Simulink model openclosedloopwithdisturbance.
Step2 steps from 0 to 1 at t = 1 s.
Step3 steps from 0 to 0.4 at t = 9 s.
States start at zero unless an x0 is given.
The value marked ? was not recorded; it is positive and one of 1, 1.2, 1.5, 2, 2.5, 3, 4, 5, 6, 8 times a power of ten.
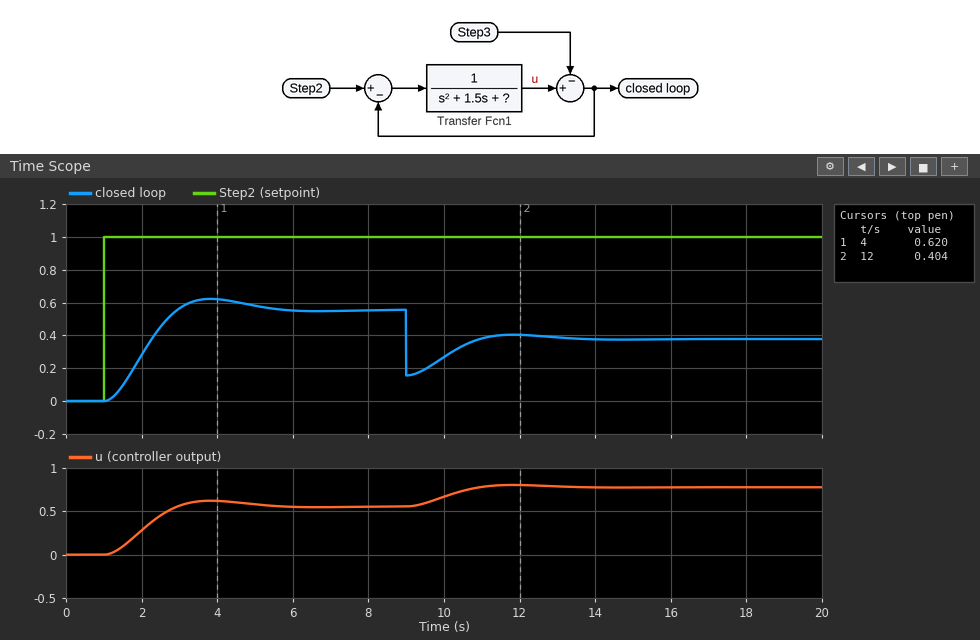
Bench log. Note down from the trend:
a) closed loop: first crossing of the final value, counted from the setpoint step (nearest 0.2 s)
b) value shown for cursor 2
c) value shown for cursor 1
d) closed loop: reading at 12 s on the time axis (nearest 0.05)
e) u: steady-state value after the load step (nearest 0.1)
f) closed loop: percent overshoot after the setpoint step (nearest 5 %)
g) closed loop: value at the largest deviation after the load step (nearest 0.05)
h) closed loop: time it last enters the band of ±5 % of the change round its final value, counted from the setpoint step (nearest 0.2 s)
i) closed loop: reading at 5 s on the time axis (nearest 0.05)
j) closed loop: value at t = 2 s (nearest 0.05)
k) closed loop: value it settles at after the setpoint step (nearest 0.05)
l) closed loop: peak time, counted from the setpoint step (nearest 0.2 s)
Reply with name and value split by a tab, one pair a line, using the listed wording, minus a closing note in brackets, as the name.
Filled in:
closed loop: first crossing of the final value, counted from the setpoint step	2.0 s
value shown for cursor 2	0.404
value shown for cursor 1	0.620
closed loop: reading at 12 s on the time axis	0.40
u: steady-state value after the load step	0.8
closed loop: percent overshoot after the setpoint step	10 %
closed loop: value at the largest deviation after the load step	0.15
closed loop: time it last enters the band of ±5 % of the change round its final value, counted from the setpoint step	4.0 s
closed loop: reading at 5 s on the time axis	0.60
closed loop: value at t = 2 s	0.30
closed loop: value it settles at after the setpoint step	0.55
closed loop: peak time, counted from the setpoint step	2.8 s
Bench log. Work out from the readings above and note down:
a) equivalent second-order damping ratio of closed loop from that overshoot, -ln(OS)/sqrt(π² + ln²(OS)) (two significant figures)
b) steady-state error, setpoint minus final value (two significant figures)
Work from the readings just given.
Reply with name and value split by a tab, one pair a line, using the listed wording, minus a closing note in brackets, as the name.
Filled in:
equivalent second-order damping ratio of closed loop from that overshoot, -ln(OS)/sqrt(π² + ln²(OS))	0.59
steady-state error, setpoint minus final value	0.45
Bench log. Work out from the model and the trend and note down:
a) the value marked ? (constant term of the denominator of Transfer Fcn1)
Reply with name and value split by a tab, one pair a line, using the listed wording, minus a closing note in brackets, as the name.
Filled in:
the value marked ?	0.8
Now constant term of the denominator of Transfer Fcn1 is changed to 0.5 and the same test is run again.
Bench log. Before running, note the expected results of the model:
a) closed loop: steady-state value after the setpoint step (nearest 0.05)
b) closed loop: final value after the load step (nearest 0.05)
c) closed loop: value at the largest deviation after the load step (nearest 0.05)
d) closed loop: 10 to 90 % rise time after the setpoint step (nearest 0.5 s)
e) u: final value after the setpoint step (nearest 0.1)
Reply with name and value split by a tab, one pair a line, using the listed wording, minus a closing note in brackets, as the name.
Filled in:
closed loop: steady-state value after the setpoint step	0.65
closed loop: final value after the load step	0.55
closed loop: value at the largest deviation after the load step	0.25
closed loop: 10 to 90 % rise time after the setpoint step	1.5 s
u: final value after the setpoint step	0.7
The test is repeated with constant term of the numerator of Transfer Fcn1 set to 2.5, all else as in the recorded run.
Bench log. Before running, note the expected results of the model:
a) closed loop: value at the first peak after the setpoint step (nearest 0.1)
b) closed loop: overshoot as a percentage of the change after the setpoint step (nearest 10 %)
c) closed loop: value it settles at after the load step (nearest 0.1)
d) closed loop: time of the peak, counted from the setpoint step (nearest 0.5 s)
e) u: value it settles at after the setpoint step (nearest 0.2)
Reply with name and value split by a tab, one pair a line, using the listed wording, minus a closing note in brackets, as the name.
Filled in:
closed loop: value at the first peak after the setpoint step	0.9
closed loop: overshoot as a percentage of the change after the setpoint step	20 %
closed loop: value it settles at after the load step	0.7
closed loop: time of the peak, counted from the setpoint step	2.0 s
u: value it settles at after the setpoint step	0.8
